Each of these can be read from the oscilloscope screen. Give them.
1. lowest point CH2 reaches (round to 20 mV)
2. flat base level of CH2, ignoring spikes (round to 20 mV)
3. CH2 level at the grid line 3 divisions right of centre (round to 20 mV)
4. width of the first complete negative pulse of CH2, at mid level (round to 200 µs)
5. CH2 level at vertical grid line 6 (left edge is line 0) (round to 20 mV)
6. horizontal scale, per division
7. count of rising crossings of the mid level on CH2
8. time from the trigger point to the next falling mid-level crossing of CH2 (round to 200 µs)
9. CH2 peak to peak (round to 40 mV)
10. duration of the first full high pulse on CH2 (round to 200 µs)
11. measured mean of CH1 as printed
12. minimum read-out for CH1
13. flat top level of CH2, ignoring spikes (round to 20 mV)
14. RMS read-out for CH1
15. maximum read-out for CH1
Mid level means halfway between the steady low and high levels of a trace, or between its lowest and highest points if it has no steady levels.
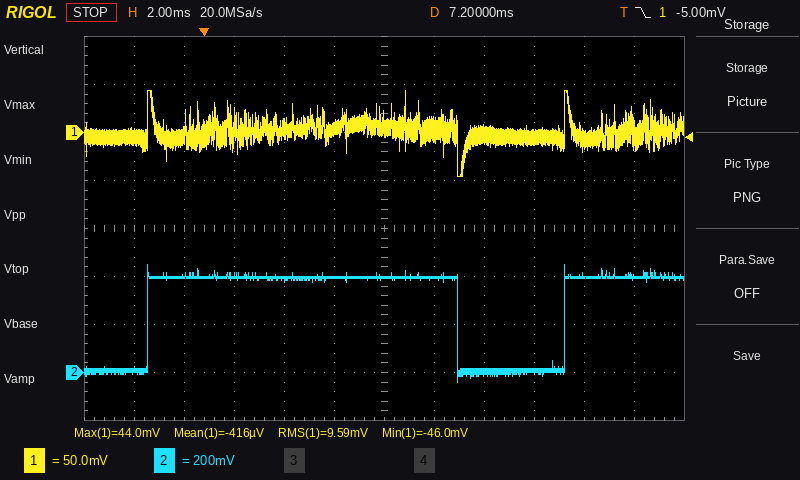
-40 mV
0 mV
0 mV
4.2 ms
400 mV
2 ms
2
10.2 ms
480 mV
12.4 ms
-416 µV
-46.0 mV
400 mV
9.59 mV
44.0 mV
